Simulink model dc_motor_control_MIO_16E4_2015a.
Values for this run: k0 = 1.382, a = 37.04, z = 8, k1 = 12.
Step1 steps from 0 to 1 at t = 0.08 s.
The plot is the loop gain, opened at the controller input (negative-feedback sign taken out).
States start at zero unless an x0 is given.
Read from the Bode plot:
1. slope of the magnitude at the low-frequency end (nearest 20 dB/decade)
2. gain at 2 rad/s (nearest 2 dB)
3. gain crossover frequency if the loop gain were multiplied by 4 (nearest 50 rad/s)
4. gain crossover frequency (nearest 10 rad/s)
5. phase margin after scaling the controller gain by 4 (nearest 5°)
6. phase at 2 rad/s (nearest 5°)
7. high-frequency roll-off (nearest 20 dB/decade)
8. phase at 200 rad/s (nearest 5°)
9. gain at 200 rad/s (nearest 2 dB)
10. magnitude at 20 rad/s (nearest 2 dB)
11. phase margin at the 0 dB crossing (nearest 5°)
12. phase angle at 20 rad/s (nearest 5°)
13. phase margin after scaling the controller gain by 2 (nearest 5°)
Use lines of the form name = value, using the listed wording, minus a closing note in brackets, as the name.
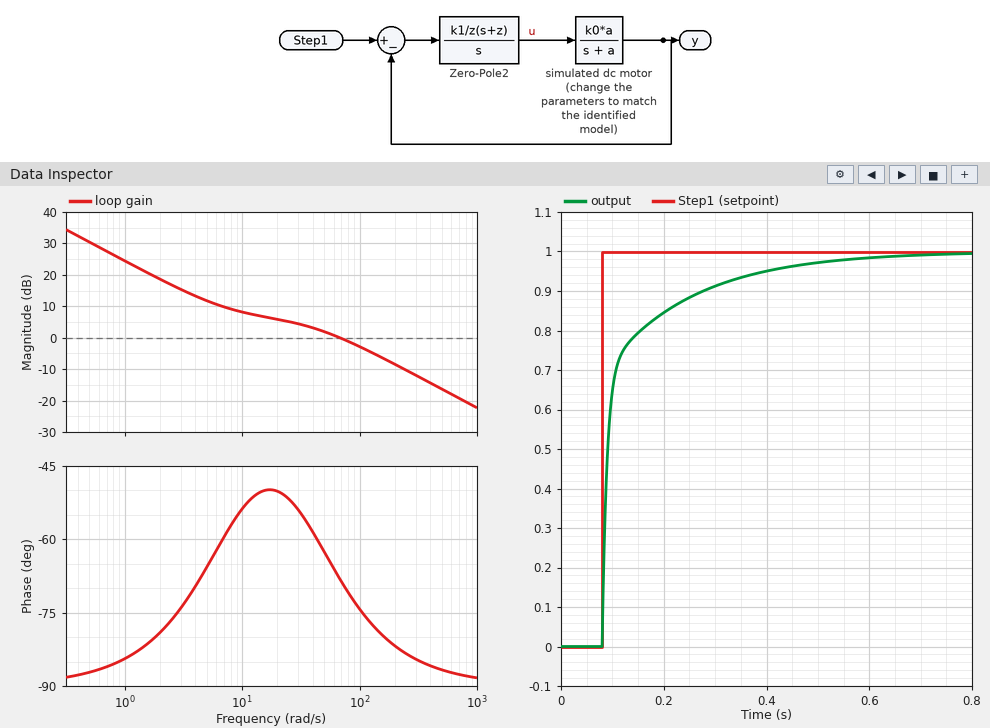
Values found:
slope of the magnitude at the low-frequency end = -20 dB/decade
gain at 2 rad/s = 18 dB
gain crossover frequency if the loop gain were multiplied by 4 = 300 rad/s
gain crossover frequency = 70 rad/s
phase margin after scaling the controller gain by 4 = 95°
phase at 2 rad/s = -80°
high-frequency roll-off = -20 dB/decade
phase at 200 rad/s = -80°
gain at 200 rad/s = -8 dB
magnitude at 20 rad/s = 6 dB
phase margin at the 0 dB crossing = 110°
phase angle at 20 rad/s = -50°
phase margin after scaling the controller gain by 2 = 100°
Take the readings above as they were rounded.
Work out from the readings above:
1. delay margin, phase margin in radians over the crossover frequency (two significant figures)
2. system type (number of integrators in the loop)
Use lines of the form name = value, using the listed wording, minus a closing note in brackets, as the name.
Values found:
delay margin, phase margin in radians over the crossover frequency = 0.027 s
system type = 1
